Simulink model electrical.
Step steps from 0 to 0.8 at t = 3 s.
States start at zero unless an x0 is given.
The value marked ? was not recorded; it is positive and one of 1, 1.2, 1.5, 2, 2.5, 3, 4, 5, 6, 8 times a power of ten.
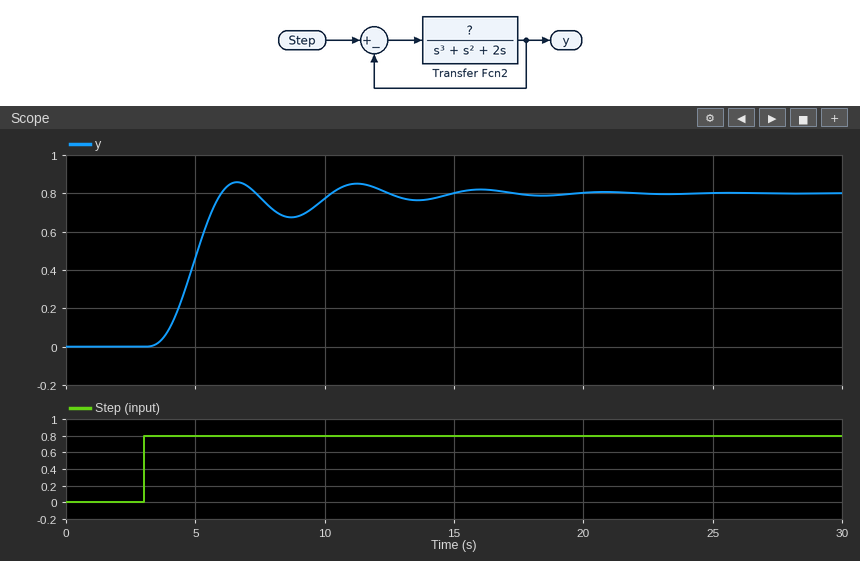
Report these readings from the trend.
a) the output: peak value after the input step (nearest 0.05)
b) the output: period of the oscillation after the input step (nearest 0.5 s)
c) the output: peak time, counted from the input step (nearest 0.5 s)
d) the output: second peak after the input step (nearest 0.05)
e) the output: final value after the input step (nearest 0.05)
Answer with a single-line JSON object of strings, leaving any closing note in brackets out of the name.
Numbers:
{"the output: peak value after the input step": "0.85", "the output: period of the oscillation after the input step": "4.5 s", "the output: peak time, counted from the input step": "3.5 s", "the output: second peak after the input step": "0.85", "the output: final value after the input step": "0.80"}
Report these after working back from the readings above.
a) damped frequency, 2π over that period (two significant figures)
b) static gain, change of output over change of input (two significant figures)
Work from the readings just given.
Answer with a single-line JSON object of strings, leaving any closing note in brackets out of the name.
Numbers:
{"damped frequency, 2π over that period": "1.4 rad/s", "static gain, change of output over change of input": "1.0"}
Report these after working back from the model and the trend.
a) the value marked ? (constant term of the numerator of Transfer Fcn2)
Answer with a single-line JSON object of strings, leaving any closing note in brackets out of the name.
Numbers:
{"the value marked ?": "1"}
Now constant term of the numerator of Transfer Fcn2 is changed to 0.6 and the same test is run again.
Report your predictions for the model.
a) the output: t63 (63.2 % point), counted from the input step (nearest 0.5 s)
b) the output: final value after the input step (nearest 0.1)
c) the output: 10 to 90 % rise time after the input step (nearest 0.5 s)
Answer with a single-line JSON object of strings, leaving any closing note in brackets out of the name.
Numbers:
{"the output: t63 (63.2 % point), counted from the input step": "3.0 s", "the output: final value after the input step": "0.8", "the output: 10 to 90 % rise time after the input step": "6.0 s"}
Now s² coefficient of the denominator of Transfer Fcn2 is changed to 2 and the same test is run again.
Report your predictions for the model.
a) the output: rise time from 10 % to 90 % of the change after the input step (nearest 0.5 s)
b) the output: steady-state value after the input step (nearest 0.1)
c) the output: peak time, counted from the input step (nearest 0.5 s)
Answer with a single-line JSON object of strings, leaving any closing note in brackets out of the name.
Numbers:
{"the output: rise time from 10 % to 90 % of the change after the input step": "2.5 s", "the output: steady-state value after the input step": "0.8", "the output: peak time, counted from the input step": "5.0 s"}
